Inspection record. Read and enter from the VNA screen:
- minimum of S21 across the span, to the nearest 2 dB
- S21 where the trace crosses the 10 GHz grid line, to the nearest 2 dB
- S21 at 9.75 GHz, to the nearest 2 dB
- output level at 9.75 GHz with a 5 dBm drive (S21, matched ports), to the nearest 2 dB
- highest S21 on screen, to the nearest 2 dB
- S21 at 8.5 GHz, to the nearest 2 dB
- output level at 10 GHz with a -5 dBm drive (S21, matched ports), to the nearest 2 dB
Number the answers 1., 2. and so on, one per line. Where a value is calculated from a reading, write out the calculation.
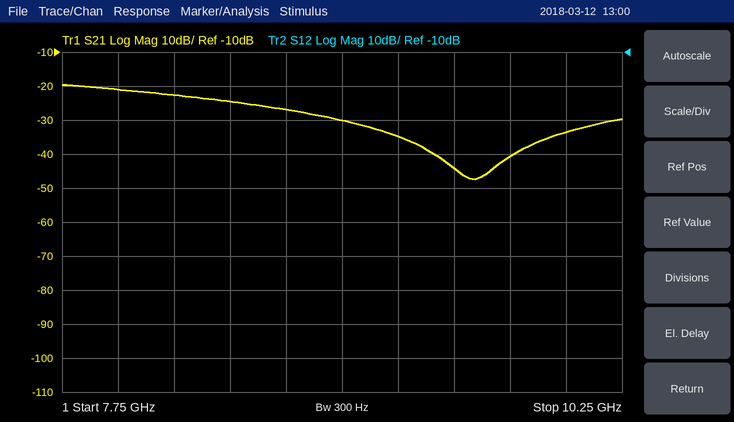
1. -48 dB
2. -34 dB
3. -40 dB
4. 5 dBm + (-40 dB) = -36 dBm
5. -20 dB
6. -24 dB
7. -5 dBm + (-34 dB) = -38 dBm
